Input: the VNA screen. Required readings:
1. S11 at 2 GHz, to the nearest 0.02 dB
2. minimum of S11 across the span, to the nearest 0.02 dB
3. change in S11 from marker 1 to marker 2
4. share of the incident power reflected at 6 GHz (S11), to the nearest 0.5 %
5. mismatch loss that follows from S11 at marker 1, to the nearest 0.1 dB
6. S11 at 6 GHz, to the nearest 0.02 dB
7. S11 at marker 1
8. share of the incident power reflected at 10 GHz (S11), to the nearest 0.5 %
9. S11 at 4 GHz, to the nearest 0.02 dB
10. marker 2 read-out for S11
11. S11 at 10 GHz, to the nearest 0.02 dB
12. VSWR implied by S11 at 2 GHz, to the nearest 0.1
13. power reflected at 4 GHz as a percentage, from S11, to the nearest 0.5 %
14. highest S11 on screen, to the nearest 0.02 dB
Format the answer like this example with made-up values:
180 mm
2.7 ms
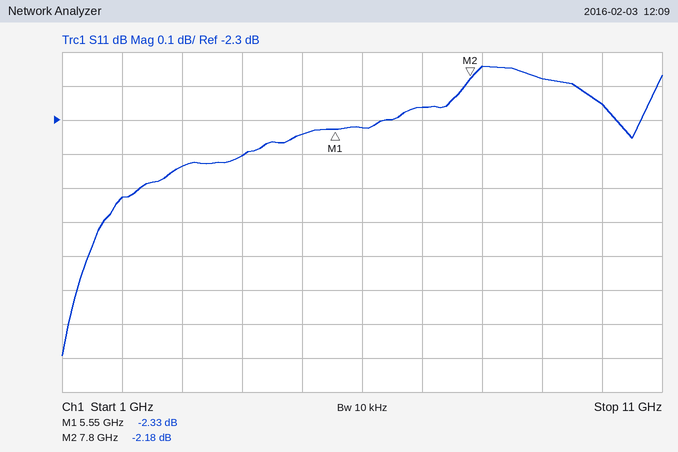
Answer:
-2.52 dB
-3.00 dB
0.15 dB
58.5 %
3.8 dB
-2.32 dB
-2.33 dB
59.5 %
-2.40 dB
-2.18 dB
-2.26 dB
6.9
57.5 %
-2.14 dB
